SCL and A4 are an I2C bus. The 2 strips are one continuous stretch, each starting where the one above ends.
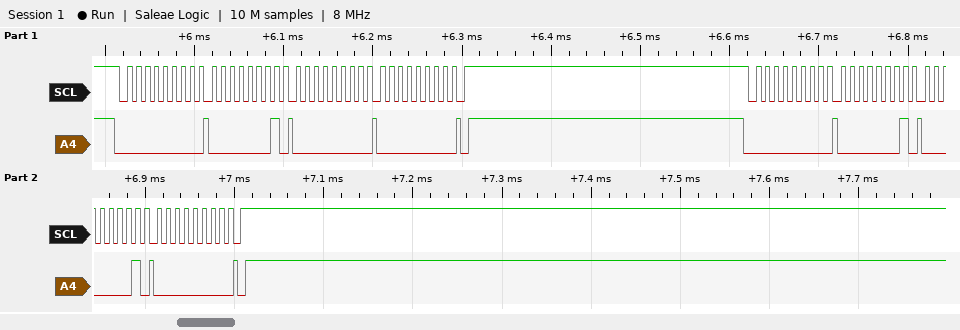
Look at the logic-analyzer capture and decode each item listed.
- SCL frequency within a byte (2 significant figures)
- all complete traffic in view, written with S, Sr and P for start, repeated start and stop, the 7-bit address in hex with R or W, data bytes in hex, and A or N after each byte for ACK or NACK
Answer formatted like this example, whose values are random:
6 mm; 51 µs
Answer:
100 kHz; S 00W A 01 A 00 A 00 A P S 00W A 01 A 01 A 00 A P
